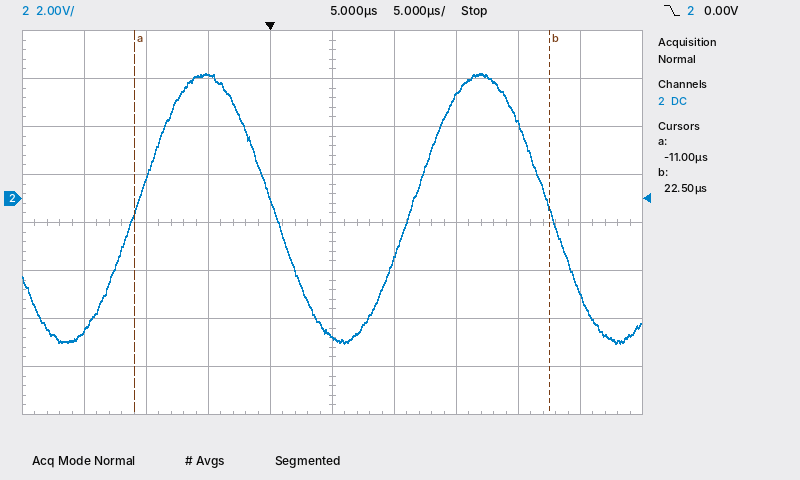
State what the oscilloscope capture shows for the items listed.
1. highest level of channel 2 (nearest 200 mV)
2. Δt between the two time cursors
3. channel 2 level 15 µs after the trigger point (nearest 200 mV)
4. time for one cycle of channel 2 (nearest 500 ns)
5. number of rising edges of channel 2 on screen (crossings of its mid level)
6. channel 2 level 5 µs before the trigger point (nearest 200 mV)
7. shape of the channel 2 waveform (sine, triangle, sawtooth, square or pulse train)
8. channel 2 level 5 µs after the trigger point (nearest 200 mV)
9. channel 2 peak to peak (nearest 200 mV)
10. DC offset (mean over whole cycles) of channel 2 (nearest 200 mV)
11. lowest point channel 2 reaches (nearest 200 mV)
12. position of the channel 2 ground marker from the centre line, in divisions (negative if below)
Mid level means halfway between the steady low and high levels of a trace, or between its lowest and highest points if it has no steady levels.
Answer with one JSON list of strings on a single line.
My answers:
["5.2 V", "33.5 µs", "4.2 V", "22.0 µs", "2", "5.2 V", "sine", "-5.8 V", "11.2 V", "-400 mV", "-6.0 V", "+0.5 div"]
